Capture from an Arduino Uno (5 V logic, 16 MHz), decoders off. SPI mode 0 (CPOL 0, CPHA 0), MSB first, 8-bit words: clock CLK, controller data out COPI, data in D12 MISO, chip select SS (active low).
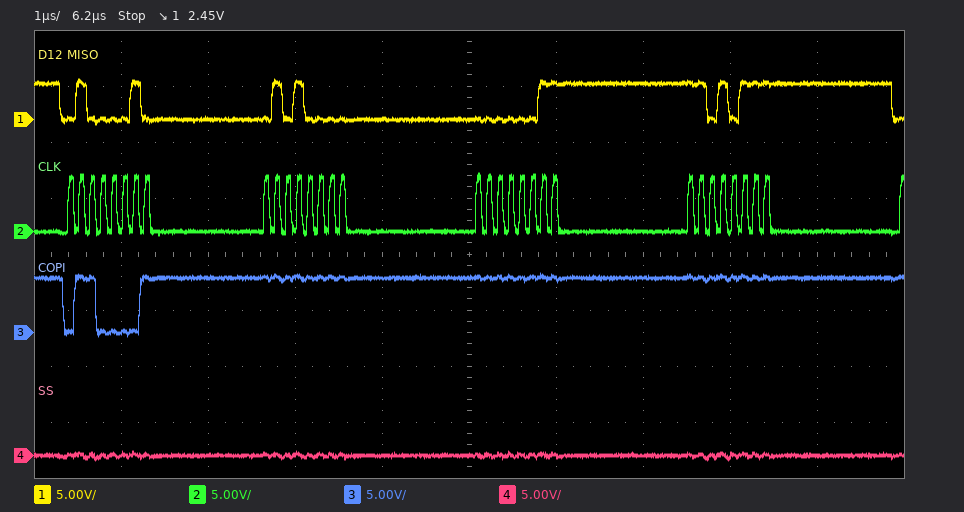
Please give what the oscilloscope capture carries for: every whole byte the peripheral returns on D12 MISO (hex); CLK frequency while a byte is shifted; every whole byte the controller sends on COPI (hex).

42 50 03 D7
8 MHz
61 FF FF FF
